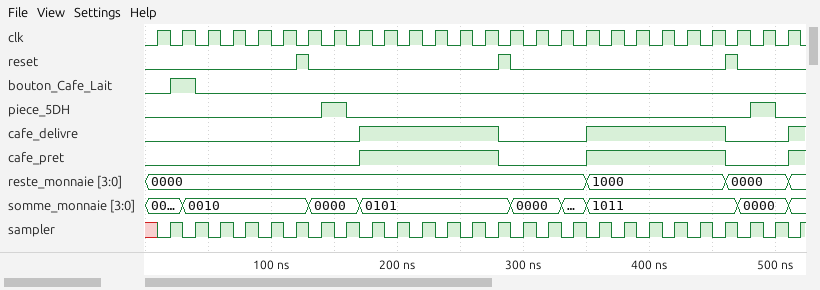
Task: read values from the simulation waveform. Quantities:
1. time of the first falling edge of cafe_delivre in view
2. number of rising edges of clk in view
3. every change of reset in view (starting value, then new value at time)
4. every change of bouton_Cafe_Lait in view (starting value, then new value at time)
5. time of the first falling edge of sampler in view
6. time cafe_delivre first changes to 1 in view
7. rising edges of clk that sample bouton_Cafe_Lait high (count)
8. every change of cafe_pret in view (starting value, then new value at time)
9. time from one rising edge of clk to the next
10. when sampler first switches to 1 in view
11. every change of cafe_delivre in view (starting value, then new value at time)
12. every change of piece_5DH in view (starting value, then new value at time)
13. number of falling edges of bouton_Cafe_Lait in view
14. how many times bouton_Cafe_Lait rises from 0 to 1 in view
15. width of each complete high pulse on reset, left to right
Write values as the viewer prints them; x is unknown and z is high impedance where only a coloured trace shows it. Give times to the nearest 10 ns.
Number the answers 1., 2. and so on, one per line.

1. 280 ns
2. 26
3. 0, 1 at 120 ns, 0 at 130 ns, 1 at 280 ns, 0 at 290 ns, 1 at 460 ns, 0 at 470 ns
4. 0, 1 at 20 ns, 0 at 40 ns
5. 30 ns
6. 170 ns
7. 1
8. 0, 1 at 170 ns, 0 at 280 ns, 1 at 350 ns, 0 at 460 ns, 1 at 510 ns
9. 20 ns
10. 20 ns
11. 0, 1 at 170 ns, 0 at 280 ns, 1 at 350 ns, 0 at 460 ns, 1 at 510 ns
12. 0, 1 at 140 ns, 0 at 160 ns, 1 at 480 ns, 0 at 500 ns
13. 1
14. 1
15. 10 ns, 10 ns, 10 ns
